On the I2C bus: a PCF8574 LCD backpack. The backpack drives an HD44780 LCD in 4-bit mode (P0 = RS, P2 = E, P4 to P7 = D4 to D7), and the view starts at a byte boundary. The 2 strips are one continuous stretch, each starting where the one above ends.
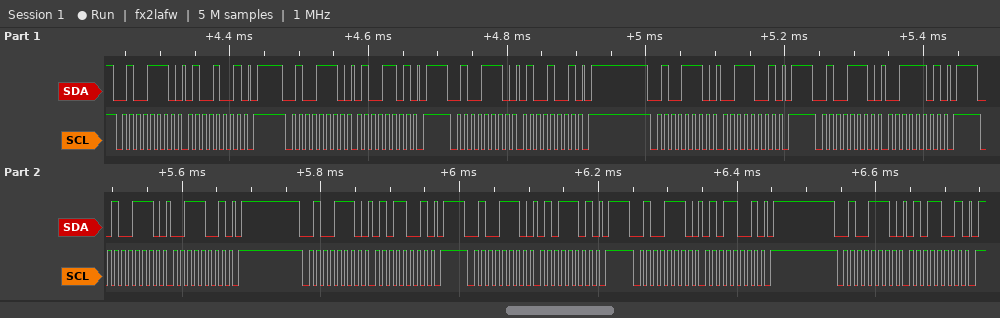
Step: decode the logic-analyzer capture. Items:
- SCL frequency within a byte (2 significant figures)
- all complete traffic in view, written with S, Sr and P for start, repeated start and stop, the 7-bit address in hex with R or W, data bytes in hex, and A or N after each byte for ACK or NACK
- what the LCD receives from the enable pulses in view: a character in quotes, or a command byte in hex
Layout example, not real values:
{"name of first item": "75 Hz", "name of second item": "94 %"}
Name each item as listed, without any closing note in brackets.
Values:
{"SCL frequency within a byte": "100 kHz", "all complete traffic in view, written with S, Sr and P for start, repeated start and stop, the 7-bit address in hex with R or W, data bytes in hex, and A or N after each byte for ACK or NACK": "S 27W A 49 A P S 27W A 4D A P S 27W A 49 A P S 27W A 39 A P S 27W A 3D A P S 27W A 39 A P S 27W A 59 A P S 27W A 5D A P S 27W A 59 A P S 27W A 59 A P", "what the LCD receives from the enable pulses in view: a character in quotes, or a command byte in hex": "'C'"}
